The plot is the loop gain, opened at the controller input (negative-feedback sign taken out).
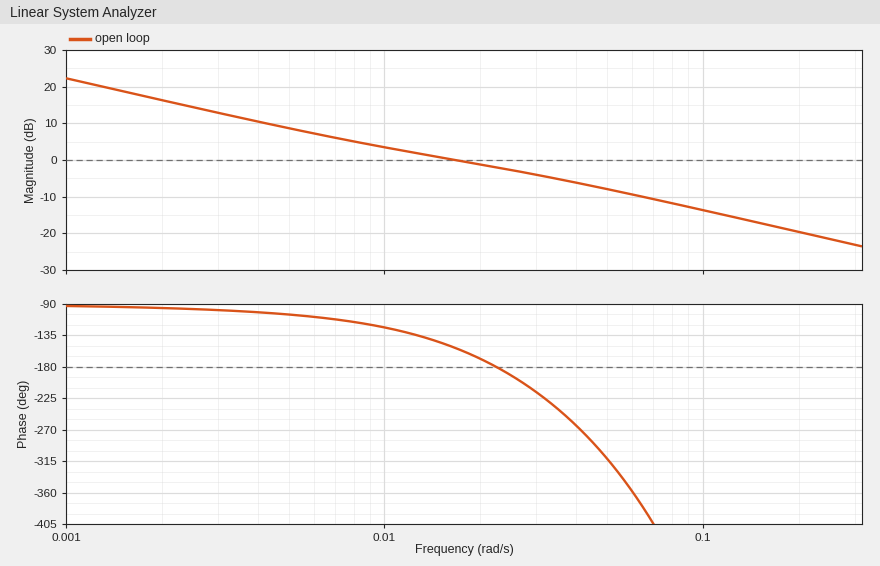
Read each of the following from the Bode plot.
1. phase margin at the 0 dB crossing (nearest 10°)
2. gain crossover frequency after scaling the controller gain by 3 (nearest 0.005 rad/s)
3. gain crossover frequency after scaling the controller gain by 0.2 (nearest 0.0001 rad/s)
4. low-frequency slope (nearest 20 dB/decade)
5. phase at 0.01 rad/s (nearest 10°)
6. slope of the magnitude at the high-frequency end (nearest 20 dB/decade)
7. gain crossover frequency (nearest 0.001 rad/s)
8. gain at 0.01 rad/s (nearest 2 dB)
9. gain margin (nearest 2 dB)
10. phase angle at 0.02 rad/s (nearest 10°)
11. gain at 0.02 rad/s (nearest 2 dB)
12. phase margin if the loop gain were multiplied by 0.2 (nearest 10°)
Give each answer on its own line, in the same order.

30°
0.060 rad/s
0.0026 rad/s
-20 dB/decade
-120°
-20 dB/decade
0.017 rad/s
4 dB
2 dB
-170°
-2 dB
80°
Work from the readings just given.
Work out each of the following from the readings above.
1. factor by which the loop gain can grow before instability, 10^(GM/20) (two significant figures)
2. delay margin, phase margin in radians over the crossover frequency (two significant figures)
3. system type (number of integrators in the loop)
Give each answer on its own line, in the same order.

1.3
31 s
1
